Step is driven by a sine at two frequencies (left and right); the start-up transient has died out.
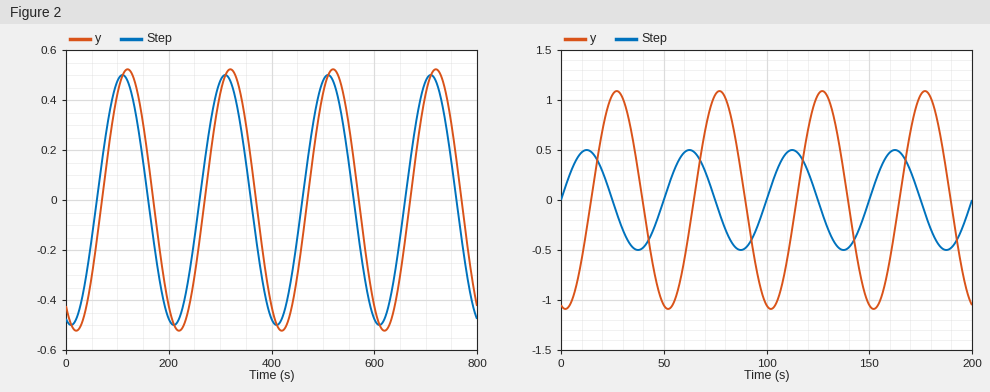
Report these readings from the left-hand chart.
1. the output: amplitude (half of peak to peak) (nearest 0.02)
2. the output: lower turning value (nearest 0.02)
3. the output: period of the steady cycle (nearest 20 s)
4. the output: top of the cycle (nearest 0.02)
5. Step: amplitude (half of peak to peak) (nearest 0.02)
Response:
0.52
-0.52
200 s
0.52
0.50
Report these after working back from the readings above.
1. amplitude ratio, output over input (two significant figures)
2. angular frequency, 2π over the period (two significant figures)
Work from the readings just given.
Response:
1.0
0.031 rad/s
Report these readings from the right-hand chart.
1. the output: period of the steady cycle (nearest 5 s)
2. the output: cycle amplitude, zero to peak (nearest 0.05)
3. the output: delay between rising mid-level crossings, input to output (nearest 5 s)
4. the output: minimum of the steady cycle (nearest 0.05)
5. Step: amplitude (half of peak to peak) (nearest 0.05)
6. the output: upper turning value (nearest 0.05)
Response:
50 s
1.10
15 s
-1.10
0.50
1.10
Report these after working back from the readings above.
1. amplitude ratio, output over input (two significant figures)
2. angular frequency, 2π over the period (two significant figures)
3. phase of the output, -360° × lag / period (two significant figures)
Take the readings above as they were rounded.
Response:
2.2
0.13 rad/s
-110°
